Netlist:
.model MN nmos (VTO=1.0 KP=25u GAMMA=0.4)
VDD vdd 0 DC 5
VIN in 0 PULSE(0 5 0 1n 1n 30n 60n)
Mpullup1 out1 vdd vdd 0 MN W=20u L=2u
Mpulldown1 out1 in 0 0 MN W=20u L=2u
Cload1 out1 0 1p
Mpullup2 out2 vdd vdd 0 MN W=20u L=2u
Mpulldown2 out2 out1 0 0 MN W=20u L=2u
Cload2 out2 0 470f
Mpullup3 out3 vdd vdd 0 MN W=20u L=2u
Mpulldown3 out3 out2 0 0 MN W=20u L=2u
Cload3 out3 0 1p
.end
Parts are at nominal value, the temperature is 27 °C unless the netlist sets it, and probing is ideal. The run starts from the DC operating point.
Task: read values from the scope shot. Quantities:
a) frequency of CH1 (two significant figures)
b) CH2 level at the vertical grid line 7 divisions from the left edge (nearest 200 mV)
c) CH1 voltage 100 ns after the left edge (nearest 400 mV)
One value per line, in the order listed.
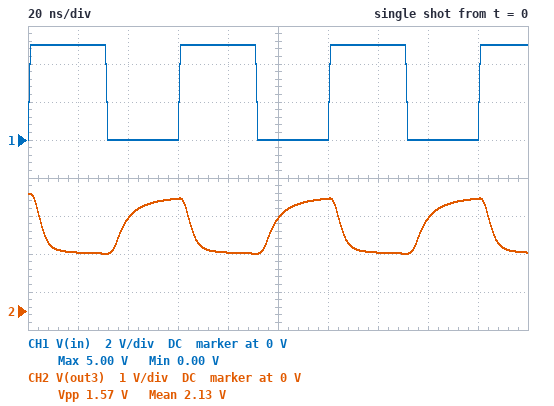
17 MHz
1.6 V
0 V
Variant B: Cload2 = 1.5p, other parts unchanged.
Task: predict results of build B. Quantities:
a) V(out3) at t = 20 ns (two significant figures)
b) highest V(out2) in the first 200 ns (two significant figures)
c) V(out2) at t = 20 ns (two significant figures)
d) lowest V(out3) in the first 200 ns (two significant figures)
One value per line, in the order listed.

1.7 V
3.2 V
3.1 V
1.6 V
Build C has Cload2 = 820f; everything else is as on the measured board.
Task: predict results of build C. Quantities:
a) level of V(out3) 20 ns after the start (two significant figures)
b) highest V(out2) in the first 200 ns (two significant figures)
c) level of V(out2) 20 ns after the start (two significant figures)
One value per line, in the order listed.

1.6 V
3.3 V
3.2 V
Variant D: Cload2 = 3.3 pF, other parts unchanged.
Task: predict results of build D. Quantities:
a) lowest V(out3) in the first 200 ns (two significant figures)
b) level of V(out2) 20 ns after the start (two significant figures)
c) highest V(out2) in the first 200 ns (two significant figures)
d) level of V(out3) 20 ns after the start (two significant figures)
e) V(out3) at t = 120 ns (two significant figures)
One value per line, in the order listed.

1.7 V
2.8 V
3.0 V
2.0 V
2.9 V
